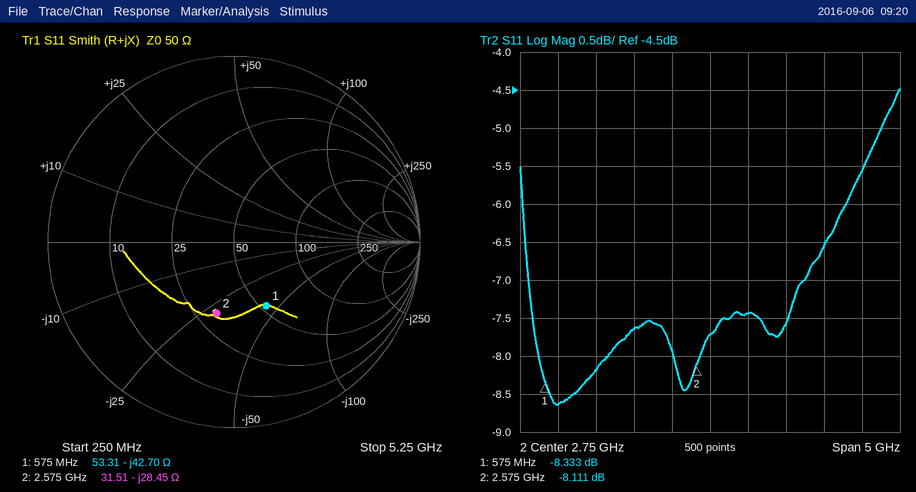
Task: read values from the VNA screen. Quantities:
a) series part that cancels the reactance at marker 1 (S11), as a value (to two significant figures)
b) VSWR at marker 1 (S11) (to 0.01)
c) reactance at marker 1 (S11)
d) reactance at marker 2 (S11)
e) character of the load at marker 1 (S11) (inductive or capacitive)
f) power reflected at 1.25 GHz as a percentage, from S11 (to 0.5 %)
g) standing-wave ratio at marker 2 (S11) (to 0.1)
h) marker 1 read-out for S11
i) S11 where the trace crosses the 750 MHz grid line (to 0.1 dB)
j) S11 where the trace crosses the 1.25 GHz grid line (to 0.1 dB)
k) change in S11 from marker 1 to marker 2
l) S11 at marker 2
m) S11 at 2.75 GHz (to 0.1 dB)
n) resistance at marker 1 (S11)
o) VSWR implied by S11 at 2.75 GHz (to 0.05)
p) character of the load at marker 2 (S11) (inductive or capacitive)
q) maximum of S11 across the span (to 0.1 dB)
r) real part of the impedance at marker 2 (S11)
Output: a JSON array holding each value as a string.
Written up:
["12 nH", "2.24", "-42.70 Ω", "-28.45 Ω", "capacitive", "15.0 %", "2.3", "-8.333 dB", "-8.6 dB", "-8.2 dB", "0.222 dB", "-8.111 dB", "-7.7 dB", "53.31 Ω", "2.40", "capacitive", "-4.5 dB", "31.51 Ω"]
